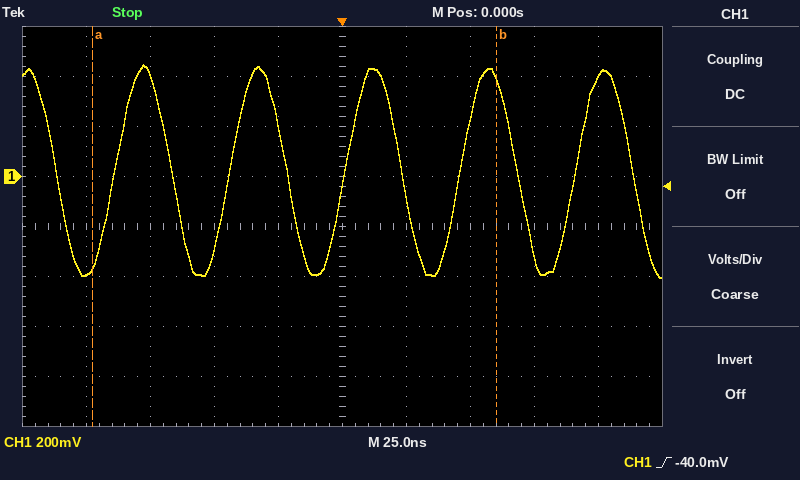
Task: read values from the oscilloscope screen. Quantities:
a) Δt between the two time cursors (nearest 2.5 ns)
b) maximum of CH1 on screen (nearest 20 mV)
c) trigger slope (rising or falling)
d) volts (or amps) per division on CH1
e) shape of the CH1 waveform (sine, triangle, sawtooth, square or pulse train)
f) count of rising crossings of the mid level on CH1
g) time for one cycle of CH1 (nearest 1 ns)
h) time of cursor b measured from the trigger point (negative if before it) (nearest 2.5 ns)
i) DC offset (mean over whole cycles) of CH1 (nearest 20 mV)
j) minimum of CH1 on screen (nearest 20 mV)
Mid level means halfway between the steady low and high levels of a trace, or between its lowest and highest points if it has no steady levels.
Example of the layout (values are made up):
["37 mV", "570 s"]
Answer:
["157.5 ns", "440 mV", "rising", "200 mV", "sine", "5", "45 ns", "+60.0 ns", "20 mV", "-400 mV"]
